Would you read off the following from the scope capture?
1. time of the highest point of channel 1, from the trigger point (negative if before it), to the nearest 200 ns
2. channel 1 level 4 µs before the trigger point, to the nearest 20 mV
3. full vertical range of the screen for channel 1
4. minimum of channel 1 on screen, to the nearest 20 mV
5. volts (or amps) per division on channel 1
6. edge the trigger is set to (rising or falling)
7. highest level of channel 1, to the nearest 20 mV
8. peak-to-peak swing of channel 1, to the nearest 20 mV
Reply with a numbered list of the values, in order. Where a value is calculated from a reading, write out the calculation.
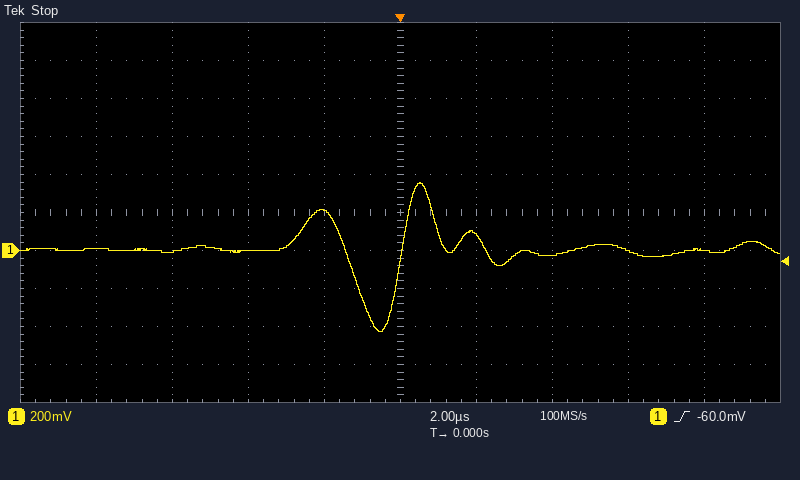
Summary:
1. +600 ns
2. 0 mV
3. 2 V
4. -420 mV
5. 200 mV
6. rising
7. 360 mV
8. 360 mV − (-420 mV) = 780 mV
